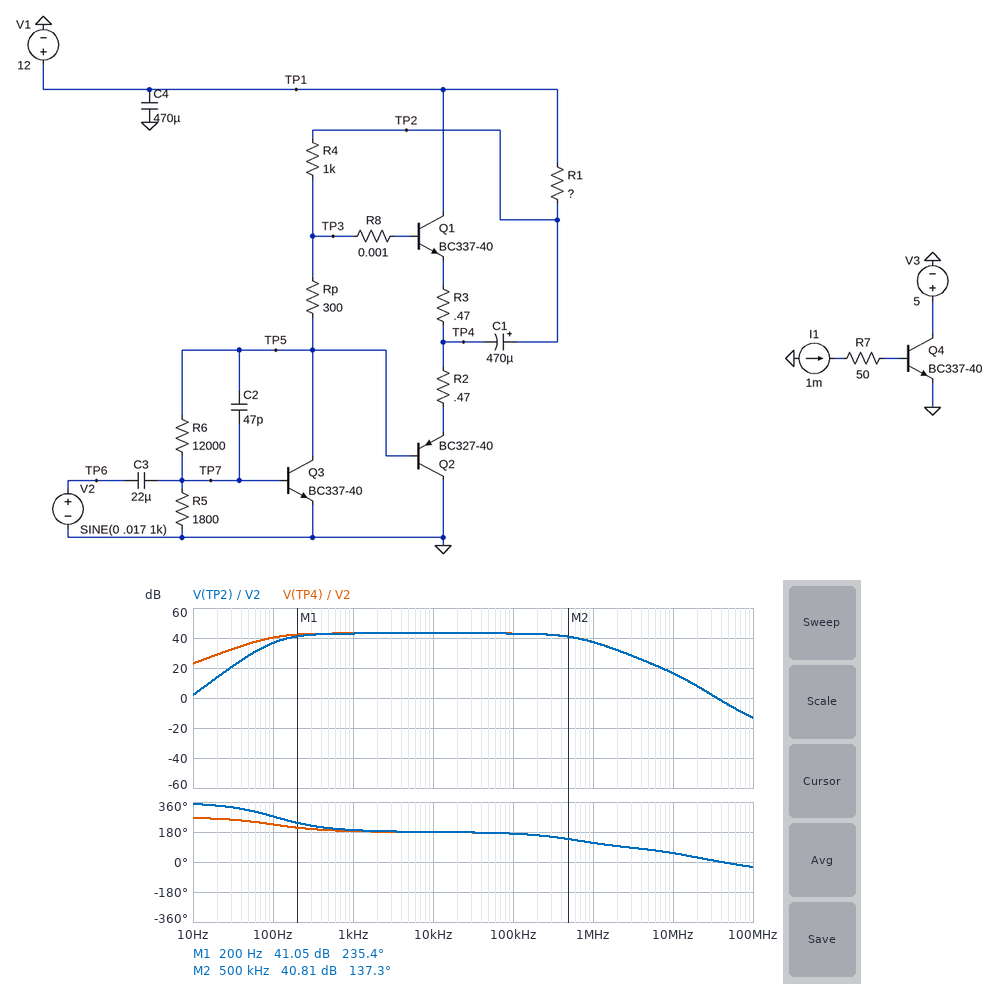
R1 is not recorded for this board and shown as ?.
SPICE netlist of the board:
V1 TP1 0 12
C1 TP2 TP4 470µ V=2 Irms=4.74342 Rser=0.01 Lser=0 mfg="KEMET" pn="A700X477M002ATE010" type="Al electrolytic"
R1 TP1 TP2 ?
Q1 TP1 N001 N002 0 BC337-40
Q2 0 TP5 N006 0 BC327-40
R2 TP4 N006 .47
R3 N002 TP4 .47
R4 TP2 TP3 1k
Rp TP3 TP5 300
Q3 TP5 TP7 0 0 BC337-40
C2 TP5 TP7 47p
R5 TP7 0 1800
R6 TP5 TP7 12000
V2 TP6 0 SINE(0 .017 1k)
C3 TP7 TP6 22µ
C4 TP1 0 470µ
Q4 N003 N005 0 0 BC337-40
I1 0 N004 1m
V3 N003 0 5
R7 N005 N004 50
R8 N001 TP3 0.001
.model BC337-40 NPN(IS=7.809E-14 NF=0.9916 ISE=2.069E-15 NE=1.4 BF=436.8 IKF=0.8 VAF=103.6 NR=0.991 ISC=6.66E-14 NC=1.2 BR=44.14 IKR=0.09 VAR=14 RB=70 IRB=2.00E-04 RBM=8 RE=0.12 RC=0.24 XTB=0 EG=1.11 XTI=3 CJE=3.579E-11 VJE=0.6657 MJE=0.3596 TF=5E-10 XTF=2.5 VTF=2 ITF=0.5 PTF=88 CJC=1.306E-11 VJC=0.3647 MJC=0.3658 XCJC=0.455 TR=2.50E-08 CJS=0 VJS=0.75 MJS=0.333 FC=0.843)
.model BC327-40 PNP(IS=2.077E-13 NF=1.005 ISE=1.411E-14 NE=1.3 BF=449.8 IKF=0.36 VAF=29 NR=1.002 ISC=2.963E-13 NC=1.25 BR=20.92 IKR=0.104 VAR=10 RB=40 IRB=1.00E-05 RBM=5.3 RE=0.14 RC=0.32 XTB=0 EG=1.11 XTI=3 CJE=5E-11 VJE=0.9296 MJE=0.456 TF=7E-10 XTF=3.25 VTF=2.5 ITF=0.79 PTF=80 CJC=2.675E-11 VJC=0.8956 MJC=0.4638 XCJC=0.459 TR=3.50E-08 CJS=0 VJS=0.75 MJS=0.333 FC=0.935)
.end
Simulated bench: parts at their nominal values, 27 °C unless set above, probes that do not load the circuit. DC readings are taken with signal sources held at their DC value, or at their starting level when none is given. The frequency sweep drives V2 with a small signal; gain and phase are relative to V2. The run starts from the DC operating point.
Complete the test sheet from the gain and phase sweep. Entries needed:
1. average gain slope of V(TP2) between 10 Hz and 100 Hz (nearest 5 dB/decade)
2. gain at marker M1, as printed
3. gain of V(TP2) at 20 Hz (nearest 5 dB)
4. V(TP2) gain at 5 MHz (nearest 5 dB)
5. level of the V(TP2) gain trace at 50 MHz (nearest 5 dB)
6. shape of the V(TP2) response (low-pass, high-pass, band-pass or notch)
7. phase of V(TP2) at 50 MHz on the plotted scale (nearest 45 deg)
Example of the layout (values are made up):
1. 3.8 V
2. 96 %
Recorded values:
1. 35 dB/decade
2. 41.05 dB
3. 15 dB
4. 25 dB
5. -5 dB
6. band-pass
7. 0 deg
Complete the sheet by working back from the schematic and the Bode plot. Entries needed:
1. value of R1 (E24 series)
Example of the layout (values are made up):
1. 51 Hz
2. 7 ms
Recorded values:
1. 3 Ω
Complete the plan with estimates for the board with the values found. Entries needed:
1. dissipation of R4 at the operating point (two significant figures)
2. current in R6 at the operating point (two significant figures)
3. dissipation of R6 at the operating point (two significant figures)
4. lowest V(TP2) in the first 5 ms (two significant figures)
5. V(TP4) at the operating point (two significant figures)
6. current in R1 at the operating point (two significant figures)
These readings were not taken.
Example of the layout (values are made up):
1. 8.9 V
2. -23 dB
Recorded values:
1. 29 mW
2. 370 µA
3. 1.6 mW
4. 10 V
5. 5.8 V
6. 5.4 mA
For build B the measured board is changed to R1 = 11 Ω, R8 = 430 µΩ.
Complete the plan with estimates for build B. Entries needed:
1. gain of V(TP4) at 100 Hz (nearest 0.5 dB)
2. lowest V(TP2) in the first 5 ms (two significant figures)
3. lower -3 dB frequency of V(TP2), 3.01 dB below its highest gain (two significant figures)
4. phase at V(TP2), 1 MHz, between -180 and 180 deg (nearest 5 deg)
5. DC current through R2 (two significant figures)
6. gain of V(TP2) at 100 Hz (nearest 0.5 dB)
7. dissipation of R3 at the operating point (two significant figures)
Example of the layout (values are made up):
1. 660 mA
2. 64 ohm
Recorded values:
1. 42.0 dB
2. 7.3 V
3. 310 Hz
4. 110 deg
5. 92 mA
6. 41.5 dB
7. 4.0 mW
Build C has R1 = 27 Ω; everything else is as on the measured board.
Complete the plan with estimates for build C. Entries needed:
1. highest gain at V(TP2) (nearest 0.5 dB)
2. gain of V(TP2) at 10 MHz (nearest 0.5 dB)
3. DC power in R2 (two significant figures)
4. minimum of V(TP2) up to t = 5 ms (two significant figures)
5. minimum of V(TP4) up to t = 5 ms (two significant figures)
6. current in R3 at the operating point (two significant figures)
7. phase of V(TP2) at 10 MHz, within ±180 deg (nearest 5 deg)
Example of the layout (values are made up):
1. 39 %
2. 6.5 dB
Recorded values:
1. 56.5 dB
2. 26.0 dB
3. 3.4 mW
4. 6.9 V
5. 910 mV
6. 85 mA
7. 60 deg
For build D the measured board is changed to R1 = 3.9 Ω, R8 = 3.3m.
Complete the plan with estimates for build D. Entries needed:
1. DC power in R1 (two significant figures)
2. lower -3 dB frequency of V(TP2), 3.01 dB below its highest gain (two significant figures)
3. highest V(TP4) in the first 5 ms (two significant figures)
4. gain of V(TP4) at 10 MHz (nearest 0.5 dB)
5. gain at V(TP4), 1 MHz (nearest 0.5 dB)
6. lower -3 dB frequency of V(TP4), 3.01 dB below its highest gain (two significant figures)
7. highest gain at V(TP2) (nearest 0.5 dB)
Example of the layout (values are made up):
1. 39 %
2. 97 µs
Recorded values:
1. 110 µW
2. 180 Hz
3. 7.7 V
4. 18.0 dB
5. 39.0 dB
6. 140 Hz
7. 45.0 dB
